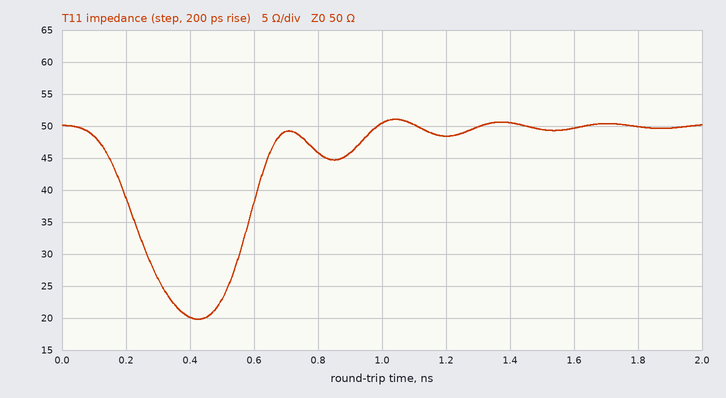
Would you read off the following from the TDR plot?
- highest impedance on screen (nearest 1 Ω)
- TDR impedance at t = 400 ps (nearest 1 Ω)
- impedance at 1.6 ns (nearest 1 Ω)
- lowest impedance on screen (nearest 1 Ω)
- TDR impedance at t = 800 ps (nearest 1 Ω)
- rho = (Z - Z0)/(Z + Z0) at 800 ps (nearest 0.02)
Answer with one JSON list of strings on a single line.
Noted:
["51 Ω", "20 Ω", "50 Ω", "20 Ω", "46 Ω", "-0.04"]
